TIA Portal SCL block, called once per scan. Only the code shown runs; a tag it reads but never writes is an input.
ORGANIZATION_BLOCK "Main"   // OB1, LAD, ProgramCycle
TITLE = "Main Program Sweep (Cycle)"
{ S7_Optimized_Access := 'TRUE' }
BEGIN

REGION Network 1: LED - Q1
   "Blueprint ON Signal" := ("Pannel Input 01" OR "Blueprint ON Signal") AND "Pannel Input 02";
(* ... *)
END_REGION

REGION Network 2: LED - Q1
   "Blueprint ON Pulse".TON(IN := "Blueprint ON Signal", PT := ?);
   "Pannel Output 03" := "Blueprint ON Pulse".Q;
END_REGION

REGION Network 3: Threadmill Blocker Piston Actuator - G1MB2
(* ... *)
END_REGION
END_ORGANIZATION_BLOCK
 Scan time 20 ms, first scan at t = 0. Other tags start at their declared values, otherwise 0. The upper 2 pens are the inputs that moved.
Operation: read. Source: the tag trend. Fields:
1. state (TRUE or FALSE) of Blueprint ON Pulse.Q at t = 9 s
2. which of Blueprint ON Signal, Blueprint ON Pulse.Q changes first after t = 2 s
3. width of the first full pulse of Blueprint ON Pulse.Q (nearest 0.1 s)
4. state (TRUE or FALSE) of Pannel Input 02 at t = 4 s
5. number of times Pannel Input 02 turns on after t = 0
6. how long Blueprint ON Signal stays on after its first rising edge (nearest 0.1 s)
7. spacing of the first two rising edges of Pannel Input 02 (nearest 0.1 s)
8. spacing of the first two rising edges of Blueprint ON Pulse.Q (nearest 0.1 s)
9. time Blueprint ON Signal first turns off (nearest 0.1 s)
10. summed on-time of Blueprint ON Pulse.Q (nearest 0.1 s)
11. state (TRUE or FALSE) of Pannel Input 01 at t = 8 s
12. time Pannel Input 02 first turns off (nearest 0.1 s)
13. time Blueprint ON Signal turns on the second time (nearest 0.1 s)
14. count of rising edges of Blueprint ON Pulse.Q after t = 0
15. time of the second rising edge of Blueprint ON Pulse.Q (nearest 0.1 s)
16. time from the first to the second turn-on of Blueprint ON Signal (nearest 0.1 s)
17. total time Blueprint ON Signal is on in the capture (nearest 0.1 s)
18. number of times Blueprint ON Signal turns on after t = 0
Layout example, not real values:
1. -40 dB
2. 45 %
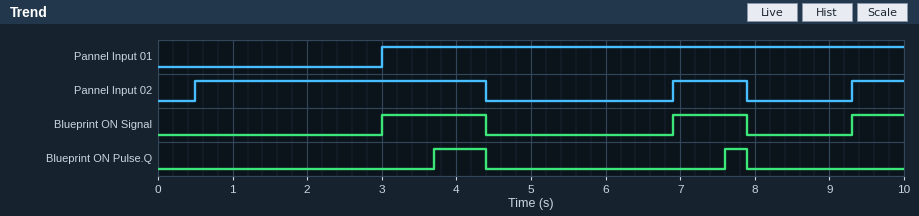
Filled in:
1. FALSE
2. Blueprint ON Signal
3. 0.7 s
4. TRUE
5. 3
6. 1.4 s
7. 6.4 s
8. 3.9 s
9. 4.4 s
10. 1.0 s
11. TRUE
12. 4.4 s
13. 6.9 s
14. 2
15. 7.6 s
16. 3.9 s
17. 3.1 s
18. 3
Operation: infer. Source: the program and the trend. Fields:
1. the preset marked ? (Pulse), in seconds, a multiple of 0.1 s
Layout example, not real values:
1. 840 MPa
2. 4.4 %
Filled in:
1. 0.7 s
